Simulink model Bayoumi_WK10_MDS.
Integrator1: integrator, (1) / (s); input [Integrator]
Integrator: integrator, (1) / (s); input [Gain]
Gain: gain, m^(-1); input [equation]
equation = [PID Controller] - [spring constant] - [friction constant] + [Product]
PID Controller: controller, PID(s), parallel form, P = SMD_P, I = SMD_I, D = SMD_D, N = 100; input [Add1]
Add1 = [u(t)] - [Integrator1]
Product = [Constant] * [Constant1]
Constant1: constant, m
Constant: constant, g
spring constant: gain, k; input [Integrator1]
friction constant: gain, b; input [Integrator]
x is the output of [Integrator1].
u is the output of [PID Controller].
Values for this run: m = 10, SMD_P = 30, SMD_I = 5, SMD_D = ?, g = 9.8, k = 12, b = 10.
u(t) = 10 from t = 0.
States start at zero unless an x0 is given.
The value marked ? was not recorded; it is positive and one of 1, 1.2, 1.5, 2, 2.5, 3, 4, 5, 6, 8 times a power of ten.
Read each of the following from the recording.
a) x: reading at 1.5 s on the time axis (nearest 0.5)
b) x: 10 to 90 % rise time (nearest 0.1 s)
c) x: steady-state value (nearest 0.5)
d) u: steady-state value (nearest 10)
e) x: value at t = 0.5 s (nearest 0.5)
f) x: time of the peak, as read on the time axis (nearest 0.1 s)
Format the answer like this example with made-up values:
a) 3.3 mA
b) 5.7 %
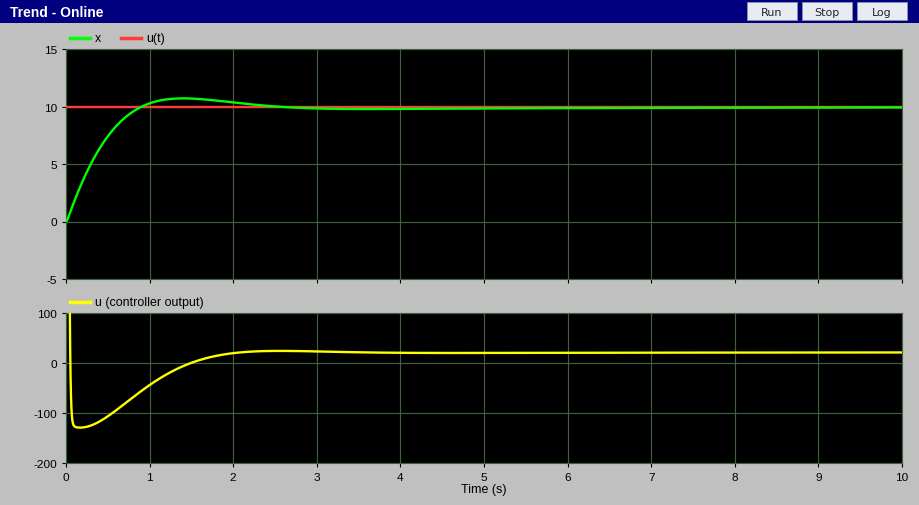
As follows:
a) 10.5
b) 0.6 s
c) 10.0
d) 20
e) 7.5
f) 1.4 s
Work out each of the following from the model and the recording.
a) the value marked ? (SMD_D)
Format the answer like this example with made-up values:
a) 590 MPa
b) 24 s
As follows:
a) 20
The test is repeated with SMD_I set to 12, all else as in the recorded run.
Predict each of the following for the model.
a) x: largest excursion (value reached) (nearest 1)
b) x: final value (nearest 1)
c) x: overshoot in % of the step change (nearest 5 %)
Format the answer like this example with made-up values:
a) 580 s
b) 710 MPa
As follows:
a) 11
b) 10
c) 10 %
